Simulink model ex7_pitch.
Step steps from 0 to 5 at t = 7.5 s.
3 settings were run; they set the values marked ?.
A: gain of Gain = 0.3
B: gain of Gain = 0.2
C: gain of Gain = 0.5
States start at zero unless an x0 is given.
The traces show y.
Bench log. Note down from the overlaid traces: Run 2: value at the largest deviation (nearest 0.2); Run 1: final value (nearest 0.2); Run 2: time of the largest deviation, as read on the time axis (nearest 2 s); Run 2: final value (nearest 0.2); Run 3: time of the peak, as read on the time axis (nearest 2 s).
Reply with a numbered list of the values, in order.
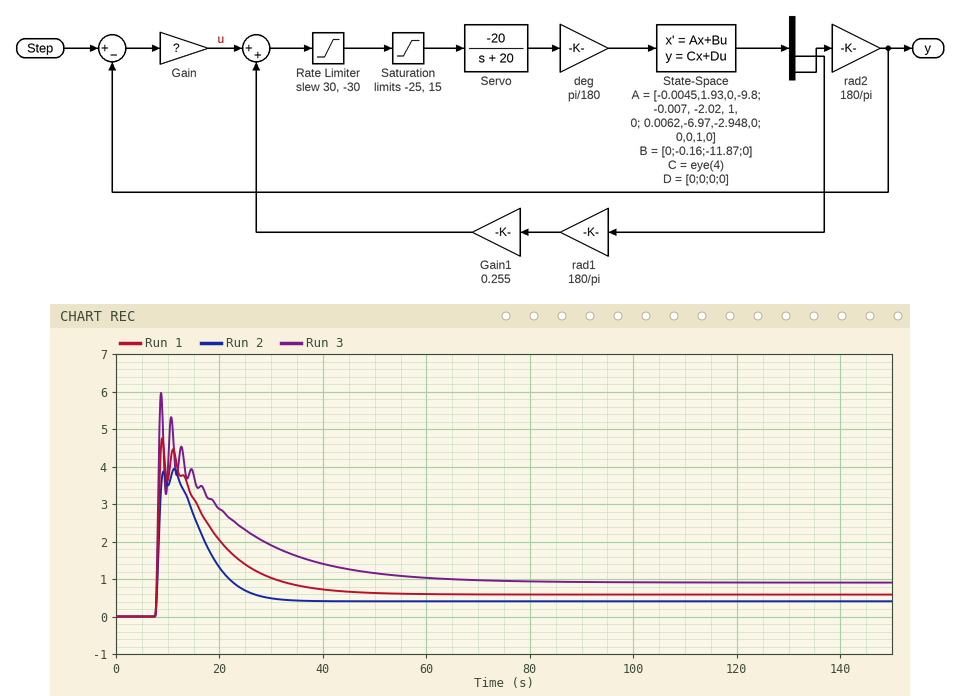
1. 4.0
2. 0.6
3. 12 s
4. 0.4
5. 8 s
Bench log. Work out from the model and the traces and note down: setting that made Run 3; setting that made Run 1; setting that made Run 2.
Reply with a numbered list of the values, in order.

1. C
2. A
3. B
